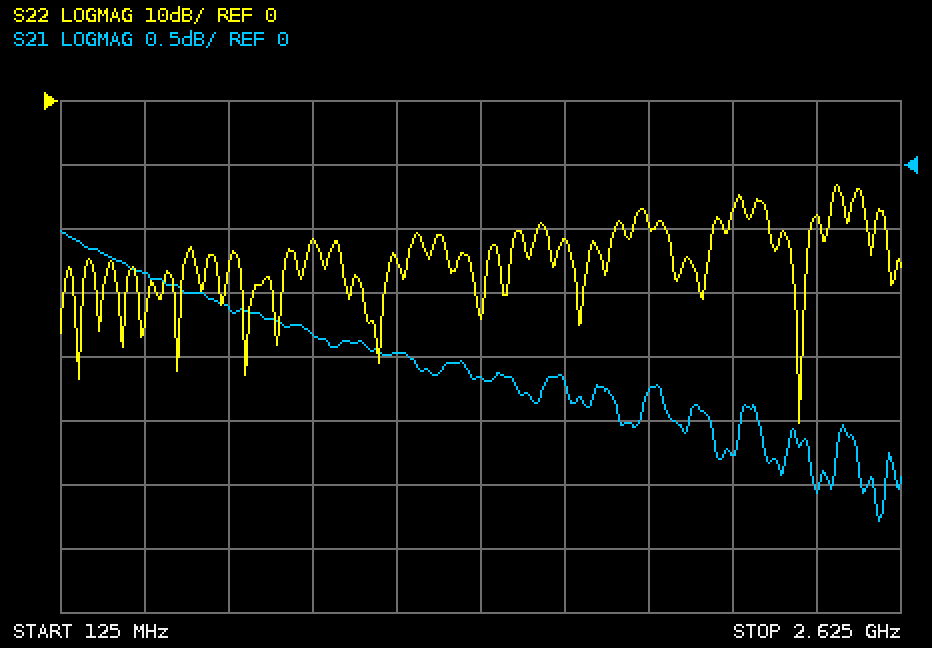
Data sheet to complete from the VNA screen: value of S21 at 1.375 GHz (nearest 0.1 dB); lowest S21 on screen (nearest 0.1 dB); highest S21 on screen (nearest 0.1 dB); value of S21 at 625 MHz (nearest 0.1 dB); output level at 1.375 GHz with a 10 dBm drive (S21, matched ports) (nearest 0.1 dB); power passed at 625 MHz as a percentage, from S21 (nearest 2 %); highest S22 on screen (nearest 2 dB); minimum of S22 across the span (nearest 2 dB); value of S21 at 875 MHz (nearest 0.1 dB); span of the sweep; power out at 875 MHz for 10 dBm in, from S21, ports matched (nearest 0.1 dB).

-1.7 dB
-2.8 dB
-0.5 dB
-1.1 dB
8.3 dBm
78 %
-14 dB
-50 dB
-1.3 dB
2.5 GHz
8.7 dBm
